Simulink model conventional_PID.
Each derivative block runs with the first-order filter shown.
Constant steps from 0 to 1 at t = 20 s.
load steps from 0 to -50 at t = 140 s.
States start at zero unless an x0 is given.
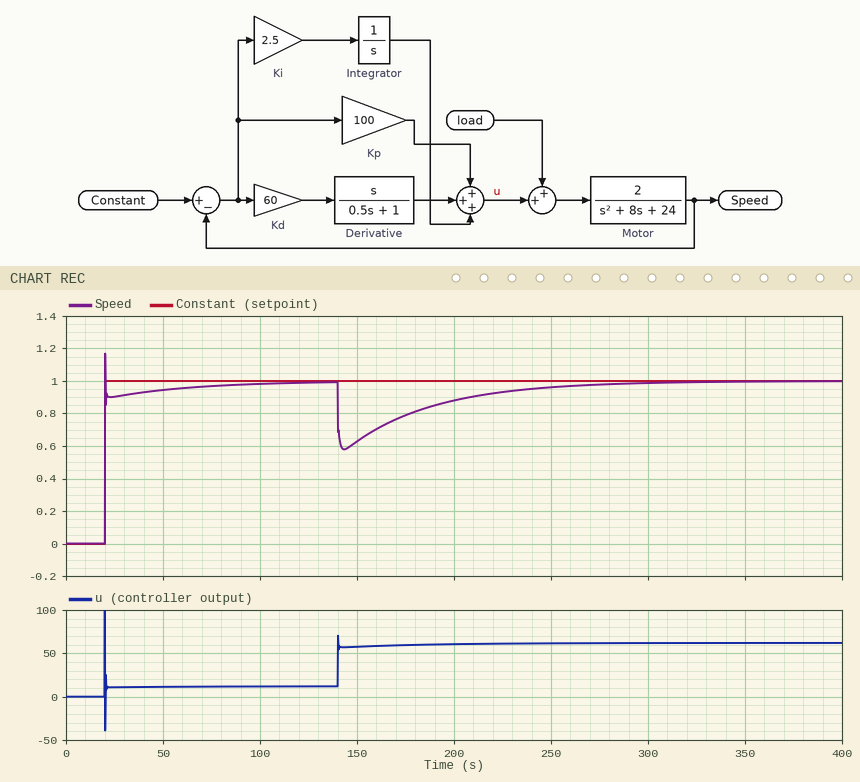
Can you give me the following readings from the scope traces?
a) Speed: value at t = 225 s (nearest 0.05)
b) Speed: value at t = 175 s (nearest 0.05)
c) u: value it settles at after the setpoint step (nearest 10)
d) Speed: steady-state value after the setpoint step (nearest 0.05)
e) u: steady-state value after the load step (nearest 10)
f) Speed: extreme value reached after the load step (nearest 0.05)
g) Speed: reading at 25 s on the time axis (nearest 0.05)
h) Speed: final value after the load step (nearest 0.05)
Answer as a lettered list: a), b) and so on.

a) 0.95
b) 0.80
c) 10
d) 1.00
e) 60
f) 0.60
g) 0.90
h) 1.00
